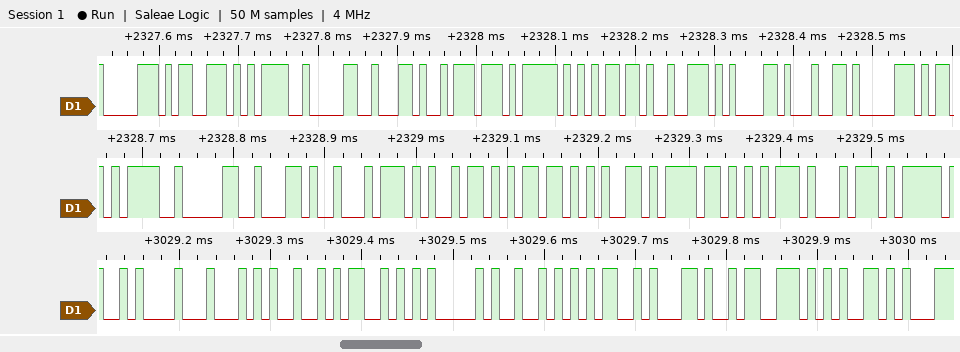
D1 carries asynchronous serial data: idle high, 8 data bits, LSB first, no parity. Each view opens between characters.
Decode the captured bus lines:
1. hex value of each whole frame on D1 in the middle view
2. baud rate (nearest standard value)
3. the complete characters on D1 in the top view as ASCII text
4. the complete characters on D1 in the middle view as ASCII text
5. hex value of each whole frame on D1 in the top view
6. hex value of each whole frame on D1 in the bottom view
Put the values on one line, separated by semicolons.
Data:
3D, 30, 2C, 74, 69, 6D, 65, 6F, 75, 74; 115200 baud; "ps=0,w_mradp"; "=0,timeout"; 70, 73, 3D, 30, 2C, 77, 5F, 6D, 72, 61, 64, 70; 0A, 44, 49, 53, 41, 52, 4D, 2C, 73, 65
